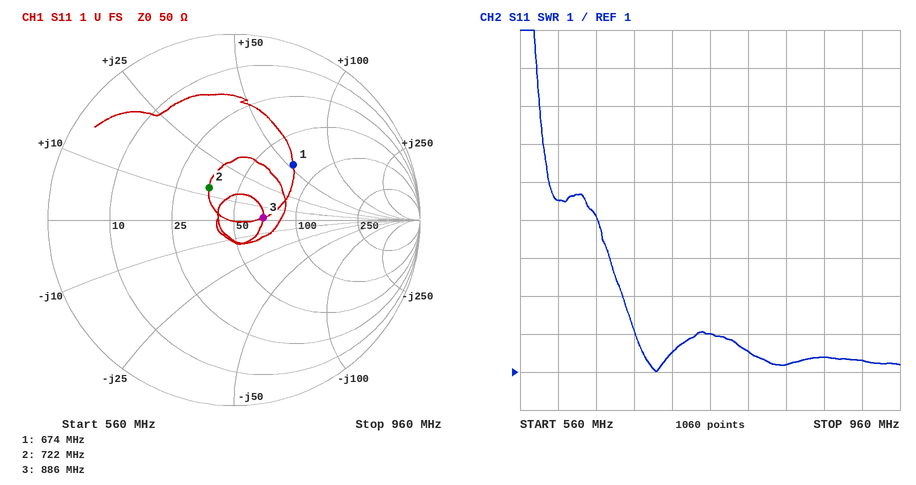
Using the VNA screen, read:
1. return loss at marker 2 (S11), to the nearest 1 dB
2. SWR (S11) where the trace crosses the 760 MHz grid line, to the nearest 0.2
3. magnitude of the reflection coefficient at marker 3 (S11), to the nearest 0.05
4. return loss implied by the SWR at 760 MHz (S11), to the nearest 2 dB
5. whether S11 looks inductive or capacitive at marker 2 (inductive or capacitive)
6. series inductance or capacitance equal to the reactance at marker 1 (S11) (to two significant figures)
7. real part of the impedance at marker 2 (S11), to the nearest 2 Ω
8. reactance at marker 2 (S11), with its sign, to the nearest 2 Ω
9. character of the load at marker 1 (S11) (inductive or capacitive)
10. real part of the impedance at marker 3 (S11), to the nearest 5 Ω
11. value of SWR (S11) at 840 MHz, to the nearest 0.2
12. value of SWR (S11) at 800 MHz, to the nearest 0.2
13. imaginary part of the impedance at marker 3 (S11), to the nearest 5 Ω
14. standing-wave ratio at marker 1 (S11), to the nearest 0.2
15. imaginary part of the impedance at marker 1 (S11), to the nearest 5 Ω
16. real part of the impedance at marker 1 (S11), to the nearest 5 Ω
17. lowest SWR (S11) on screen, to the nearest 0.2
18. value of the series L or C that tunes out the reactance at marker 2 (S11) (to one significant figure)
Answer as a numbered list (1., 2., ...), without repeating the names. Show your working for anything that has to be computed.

1. 13 dB
2. 2.0
3. 0.15
4. −20 log10((2 − 1)/(2 + 1)) ≈ 10 dB
5. inductive
6. L = 55 Ω/(2π × 674 MHz) ≈ 13 nH
7. 36 Ω
8. +14 Ω
9. inductive
10. 70 Ω
11. 1.2
12. 1.6
13. 0 Ω
14. 2.6
15. +55 Ω
16. 75 Ω
17. 1.0
18. C = 1/(2π × 722 MHz × 14 Ω) ≈ 15.7 pF, so 20 pF to one significant figure
